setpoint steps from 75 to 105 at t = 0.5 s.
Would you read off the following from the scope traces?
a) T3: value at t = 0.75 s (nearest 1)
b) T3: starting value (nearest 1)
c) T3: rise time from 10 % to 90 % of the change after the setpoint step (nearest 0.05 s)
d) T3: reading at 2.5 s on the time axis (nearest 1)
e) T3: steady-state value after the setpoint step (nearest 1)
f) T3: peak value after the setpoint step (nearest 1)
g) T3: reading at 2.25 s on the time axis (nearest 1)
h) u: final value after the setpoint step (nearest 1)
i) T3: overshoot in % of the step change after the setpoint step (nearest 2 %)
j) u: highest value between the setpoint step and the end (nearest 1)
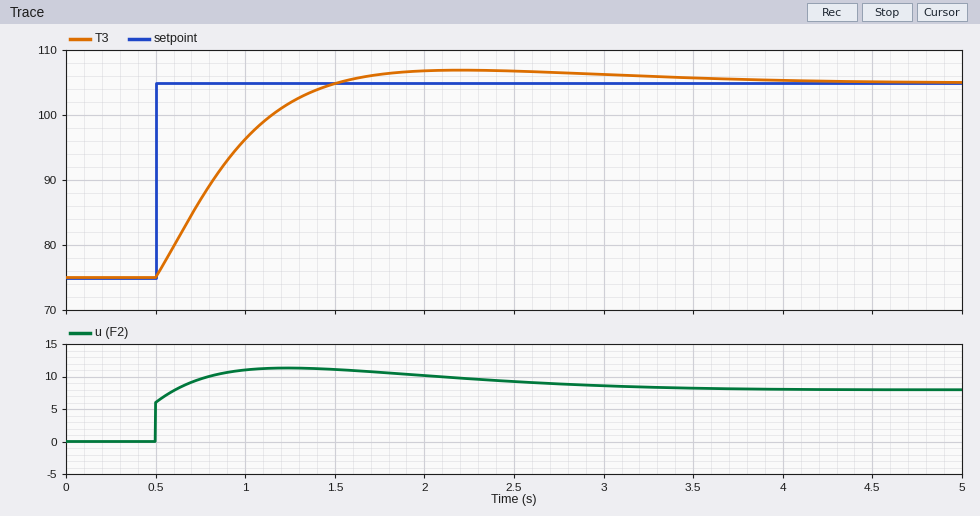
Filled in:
87
75
0.70 s
107
105
107
107
8
6 %
11
